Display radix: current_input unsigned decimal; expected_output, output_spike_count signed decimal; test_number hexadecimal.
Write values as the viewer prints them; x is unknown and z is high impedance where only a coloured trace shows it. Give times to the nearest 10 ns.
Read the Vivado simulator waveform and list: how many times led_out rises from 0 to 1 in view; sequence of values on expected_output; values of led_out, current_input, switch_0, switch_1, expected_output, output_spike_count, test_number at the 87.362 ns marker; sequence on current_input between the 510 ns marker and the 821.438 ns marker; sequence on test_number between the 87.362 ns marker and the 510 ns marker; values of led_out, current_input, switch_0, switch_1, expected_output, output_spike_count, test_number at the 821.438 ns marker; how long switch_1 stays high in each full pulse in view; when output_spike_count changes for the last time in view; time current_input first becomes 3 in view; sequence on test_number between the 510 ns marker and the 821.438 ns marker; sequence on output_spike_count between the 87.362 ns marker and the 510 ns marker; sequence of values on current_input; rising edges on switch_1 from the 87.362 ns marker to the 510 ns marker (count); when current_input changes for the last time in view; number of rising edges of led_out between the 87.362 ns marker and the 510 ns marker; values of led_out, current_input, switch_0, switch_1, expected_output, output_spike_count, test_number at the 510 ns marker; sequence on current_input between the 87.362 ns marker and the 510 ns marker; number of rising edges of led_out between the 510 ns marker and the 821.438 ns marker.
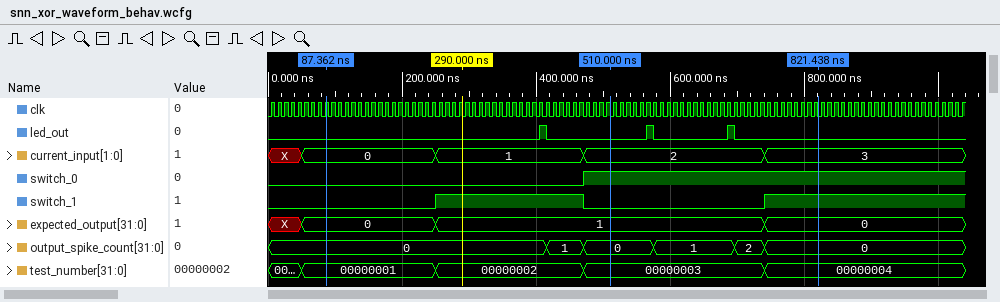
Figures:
3
X, 0, 1, 0
led_out=0, current_input=0, switch_0=0, switch_1=0, expected_output=0, output_spike_count=0, test_number=00000001
2, 3
00000001, 00000002, 00000003
led_out=0, current_input=3, switch_0=1, switch_1=1, expected_output=0, output_spike_count=0, test_number=00000004
220 ns
740 ns
740 ns
00000003, 00000004
0, 1, 0
X, 0, 1, 2, 3
1
740 ns
1
led_out=0, current_input=2, switch_0=1, switch_1=0, expected_output=1, output_spike_count=0, test_number=00000003
0, 1, 2
2
